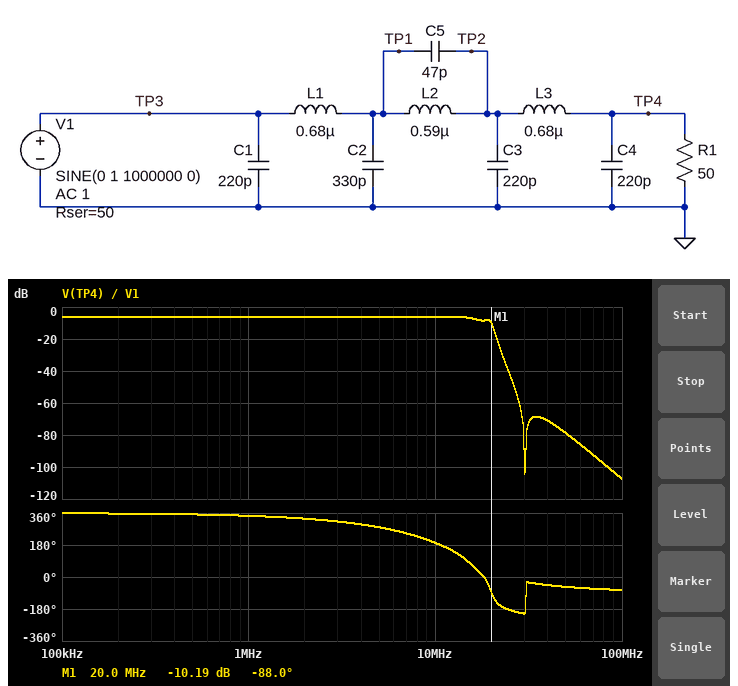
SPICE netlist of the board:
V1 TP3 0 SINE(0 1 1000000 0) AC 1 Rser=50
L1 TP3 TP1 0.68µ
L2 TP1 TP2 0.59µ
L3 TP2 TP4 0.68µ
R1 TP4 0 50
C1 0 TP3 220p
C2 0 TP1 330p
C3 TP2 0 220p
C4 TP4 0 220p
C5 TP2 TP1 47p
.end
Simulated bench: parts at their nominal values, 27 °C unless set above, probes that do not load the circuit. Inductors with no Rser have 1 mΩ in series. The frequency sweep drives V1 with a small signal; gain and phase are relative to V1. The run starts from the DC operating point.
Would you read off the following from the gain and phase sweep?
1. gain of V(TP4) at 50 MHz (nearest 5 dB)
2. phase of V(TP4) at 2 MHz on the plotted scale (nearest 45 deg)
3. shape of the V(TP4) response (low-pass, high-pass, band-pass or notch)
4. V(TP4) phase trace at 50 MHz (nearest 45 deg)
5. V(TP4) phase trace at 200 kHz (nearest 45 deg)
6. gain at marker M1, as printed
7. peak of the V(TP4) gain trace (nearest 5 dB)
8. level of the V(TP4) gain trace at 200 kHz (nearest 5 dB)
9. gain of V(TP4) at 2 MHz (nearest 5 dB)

-80 dB
315 deg
low-pass
-45 deg
360 deg
-10.19 dB
-5 dB
-5 dB
-5 dB
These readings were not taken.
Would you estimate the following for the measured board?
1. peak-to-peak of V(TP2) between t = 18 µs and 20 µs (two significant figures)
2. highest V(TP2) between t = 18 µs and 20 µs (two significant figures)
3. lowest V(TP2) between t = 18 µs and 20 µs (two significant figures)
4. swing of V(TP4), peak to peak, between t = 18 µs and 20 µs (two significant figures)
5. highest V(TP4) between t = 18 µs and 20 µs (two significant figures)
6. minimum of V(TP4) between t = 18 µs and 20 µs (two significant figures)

1.0 V
500 mV
-500 mV
1.0 V
500 mV
-500 mV
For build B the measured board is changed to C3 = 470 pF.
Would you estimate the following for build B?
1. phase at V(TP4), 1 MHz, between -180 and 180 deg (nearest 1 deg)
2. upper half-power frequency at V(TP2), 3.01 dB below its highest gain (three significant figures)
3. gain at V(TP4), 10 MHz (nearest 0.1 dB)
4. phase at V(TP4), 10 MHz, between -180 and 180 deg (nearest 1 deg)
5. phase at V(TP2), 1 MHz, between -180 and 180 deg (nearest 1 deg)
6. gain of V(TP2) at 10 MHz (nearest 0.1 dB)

-18 deg
17.7 MHz
-6.2 dB
170 deg
-13 deg
-6.6 dB
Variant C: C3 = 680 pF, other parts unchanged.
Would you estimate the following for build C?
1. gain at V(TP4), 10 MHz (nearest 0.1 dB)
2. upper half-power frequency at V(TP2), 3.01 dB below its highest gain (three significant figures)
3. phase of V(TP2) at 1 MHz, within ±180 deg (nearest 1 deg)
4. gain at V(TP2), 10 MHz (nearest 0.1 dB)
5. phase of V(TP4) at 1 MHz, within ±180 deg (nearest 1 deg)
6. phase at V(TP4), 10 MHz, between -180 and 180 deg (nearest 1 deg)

-6.9 dB
16.8 MHz
-15 deg
-7.4 dB
-20 deg
152 deg
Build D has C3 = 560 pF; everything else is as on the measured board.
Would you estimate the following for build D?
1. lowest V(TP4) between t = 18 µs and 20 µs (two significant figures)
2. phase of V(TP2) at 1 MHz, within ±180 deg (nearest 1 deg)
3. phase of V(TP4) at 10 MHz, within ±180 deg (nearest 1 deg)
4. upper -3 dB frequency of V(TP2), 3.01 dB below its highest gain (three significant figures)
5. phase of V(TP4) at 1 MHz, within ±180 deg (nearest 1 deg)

-500 mV
-14 deg
162 deg
17.4 MHz
-19 deg
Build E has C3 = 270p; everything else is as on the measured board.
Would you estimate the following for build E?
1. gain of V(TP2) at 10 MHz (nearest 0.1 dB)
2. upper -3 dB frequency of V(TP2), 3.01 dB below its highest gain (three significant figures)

-6.7 dB
19.3 MHz
